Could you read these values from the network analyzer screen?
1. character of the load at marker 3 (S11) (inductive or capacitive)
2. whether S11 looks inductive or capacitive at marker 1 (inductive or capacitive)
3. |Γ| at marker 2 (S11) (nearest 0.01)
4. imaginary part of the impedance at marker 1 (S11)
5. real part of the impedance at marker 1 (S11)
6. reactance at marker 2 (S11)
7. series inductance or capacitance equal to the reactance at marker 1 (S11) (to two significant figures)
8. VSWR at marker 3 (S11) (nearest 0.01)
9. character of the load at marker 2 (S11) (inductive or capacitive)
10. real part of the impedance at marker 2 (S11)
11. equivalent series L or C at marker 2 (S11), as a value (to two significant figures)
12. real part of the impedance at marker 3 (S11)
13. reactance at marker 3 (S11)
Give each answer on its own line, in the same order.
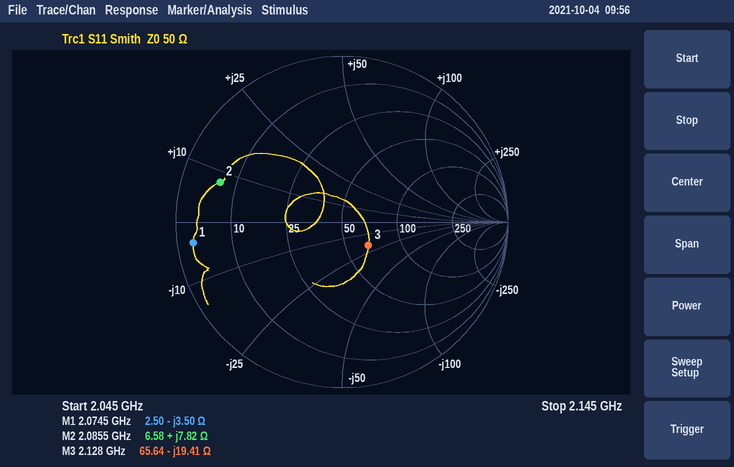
capacitive
capacitive
0.77
-3.50 Ω
2.50 Ω
+7.82 Ω
22 pF
1.54
inductive
6.58 Ω
600 pH
65.64 Ω
-19.41 Ω
